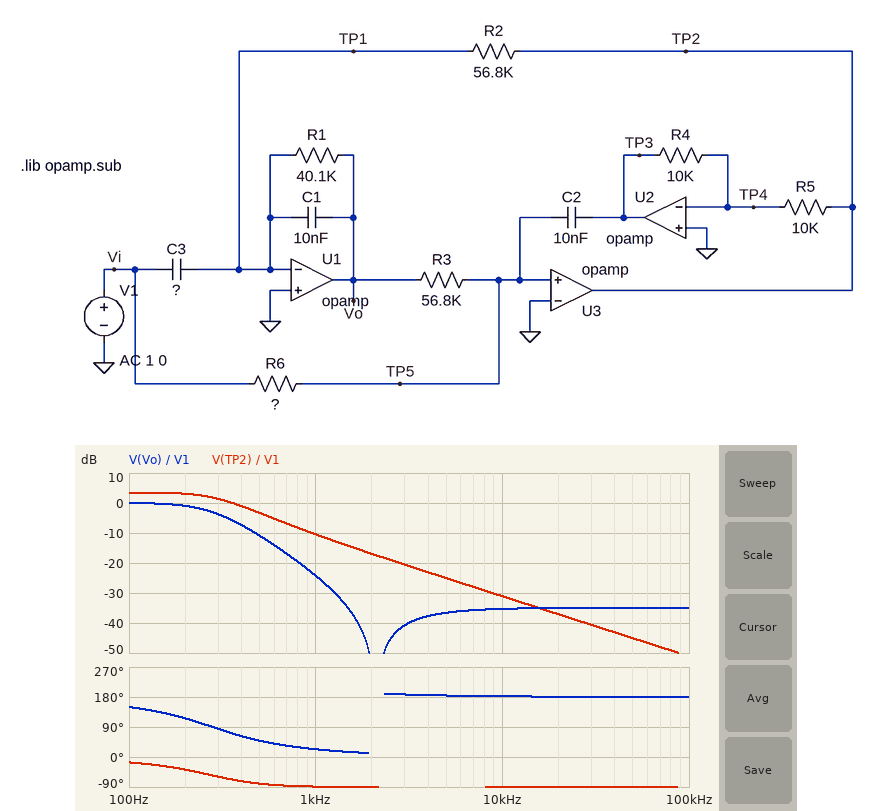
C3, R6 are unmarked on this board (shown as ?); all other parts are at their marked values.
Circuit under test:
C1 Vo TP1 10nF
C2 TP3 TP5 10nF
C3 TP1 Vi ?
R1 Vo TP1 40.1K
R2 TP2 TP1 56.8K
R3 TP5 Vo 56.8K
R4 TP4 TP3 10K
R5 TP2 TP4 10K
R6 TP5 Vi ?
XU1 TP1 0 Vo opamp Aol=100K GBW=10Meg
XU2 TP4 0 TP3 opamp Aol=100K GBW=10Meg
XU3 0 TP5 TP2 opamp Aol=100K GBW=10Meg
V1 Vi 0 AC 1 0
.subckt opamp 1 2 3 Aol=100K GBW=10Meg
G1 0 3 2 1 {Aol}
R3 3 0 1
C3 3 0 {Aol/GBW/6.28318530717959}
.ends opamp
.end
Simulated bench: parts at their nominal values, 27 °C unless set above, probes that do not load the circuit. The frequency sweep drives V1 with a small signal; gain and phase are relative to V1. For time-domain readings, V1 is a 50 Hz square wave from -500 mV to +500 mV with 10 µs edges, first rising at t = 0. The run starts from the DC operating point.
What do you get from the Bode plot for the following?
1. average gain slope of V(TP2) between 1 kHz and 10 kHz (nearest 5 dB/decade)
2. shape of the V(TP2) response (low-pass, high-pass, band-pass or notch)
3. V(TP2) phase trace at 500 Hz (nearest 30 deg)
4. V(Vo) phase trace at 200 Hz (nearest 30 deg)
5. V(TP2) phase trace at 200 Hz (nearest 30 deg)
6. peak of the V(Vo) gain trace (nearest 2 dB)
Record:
-20 dB/decade
low-pass
-90 deg
120 deg
-30 deg
0 dB
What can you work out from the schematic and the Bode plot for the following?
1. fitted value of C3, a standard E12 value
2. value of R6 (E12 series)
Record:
180 pF
56 kΩ
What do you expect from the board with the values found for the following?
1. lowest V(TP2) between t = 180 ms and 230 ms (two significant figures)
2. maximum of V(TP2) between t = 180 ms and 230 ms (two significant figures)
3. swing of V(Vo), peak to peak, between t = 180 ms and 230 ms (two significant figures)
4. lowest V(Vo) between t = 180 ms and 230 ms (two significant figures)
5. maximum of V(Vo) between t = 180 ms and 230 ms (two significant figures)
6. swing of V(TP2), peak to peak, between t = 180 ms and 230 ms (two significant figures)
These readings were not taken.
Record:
-810 mV
810 mV
1.1 V
-550 mV
550 mV
1.6 V
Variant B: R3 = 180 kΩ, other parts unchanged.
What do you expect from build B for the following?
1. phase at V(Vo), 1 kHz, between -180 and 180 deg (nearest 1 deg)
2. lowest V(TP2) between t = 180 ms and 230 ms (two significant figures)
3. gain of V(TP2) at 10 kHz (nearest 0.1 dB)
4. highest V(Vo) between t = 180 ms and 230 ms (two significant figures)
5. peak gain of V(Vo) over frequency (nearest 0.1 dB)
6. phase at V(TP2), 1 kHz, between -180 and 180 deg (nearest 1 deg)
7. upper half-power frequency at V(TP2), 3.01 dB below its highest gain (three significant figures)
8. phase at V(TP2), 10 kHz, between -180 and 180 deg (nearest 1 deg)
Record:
22 deg
-2.2 V
-31.0 dB
1.6 V
10.1 dB
-90 deg
76.1 Hz
-90 deg
